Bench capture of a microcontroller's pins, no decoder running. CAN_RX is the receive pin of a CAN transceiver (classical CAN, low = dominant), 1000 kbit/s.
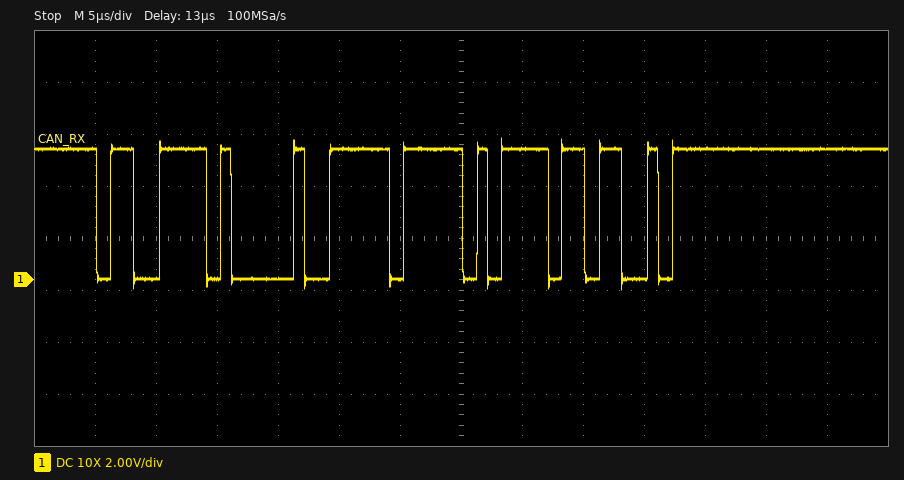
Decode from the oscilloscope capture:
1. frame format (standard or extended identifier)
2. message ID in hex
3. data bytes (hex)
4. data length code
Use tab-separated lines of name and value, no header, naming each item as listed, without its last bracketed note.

frame format	standard
message ID in hex	0x67A
data bytes	FF
data length code	1
